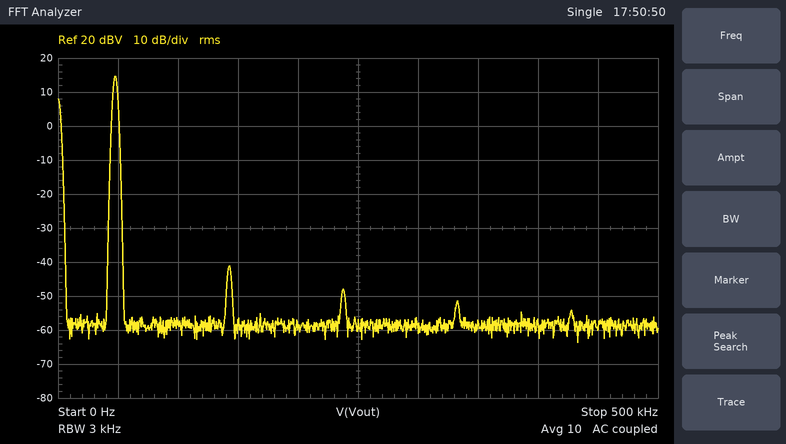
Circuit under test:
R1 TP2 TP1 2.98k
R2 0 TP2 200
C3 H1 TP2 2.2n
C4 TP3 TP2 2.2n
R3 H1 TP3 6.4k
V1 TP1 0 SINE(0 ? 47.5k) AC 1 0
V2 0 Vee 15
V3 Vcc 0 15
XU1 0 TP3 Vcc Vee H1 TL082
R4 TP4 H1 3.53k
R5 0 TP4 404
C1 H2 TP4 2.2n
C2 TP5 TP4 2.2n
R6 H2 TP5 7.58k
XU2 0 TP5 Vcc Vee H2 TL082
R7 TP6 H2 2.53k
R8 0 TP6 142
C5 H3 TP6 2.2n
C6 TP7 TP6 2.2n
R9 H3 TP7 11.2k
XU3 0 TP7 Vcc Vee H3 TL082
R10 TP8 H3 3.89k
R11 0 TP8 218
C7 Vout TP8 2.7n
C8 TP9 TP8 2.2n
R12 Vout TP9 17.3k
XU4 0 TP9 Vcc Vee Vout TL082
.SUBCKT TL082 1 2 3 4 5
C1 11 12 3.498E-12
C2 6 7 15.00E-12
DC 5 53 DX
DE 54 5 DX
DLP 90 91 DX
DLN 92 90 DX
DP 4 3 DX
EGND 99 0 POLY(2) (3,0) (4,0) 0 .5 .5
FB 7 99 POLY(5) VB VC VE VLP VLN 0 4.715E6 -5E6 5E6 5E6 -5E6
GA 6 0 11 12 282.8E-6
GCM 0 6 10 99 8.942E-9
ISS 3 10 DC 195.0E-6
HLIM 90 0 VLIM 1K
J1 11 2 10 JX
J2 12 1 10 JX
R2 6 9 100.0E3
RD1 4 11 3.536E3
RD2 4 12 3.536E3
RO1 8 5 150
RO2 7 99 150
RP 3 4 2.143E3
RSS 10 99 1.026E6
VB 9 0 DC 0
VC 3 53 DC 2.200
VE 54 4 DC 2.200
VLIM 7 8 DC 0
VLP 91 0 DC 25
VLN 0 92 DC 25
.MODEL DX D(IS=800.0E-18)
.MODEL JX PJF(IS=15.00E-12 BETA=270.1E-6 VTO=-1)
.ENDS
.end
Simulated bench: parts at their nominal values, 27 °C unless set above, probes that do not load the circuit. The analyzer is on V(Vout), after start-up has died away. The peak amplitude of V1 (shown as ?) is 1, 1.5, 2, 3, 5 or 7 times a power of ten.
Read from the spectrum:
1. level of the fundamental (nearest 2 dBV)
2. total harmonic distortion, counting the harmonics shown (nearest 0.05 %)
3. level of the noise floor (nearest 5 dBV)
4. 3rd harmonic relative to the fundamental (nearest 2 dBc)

14 dBV
0.15 %
-60 dBV
-56 dBc
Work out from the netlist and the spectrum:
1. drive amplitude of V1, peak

20 V
